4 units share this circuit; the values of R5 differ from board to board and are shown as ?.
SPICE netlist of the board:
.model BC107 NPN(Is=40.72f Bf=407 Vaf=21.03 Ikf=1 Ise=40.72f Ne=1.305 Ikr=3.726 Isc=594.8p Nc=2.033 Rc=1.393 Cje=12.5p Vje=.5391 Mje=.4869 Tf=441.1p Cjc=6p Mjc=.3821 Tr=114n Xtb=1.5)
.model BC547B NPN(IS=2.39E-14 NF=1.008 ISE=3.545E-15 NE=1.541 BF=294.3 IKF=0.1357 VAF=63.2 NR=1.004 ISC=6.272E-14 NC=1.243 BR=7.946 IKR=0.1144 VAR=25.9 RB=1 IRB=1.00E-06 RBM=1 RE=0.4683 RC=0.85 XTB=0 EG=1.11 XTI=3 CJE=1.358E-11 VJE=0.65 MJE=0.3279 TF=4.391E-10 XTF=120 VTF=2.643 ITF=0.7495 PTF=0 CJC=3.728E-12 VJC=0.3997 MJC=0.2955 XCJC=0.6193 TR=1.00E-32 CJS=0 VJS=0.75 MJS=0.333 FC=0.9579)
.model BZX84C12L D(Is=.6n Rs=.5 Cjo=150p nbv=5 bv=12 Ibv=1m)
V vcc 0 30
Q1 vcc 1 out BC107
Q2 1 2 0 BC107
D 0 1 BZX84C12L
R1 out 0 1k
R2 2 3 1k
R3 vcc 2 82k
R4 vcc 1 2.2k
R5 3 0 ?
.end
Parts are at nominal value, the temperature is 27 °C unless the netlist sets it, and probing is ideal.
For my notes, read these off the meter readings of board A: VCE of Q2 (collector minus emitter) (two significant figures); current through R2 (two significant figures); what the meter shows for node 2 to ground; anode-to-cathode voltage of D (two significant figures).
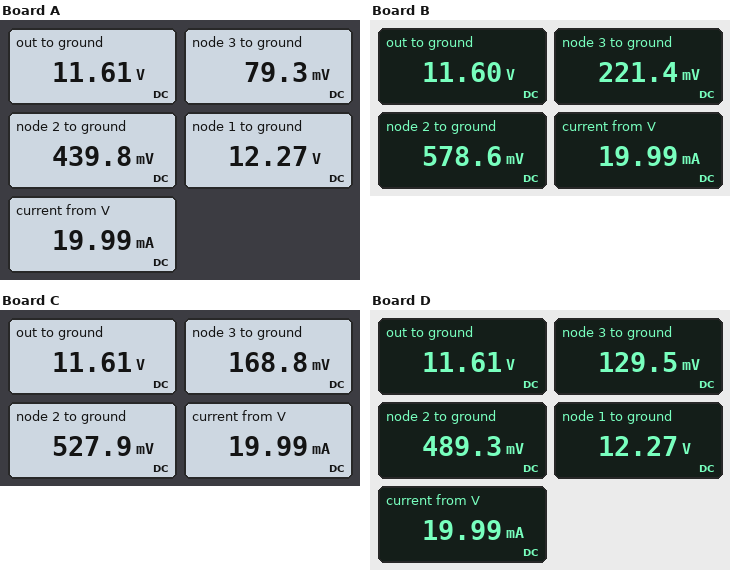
12 V
360 µA
439.8 mV
-12 V
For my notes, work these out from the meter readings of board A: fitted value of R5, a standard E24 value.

220 Ω
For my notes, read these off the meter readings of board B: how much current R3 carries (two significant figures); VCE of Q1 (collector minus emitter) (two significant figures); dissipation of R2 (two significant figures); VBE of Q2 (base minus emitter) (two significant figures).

360 µA
18 V
130 µW
580 mV
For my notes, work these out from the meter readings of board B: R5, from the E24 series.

620 Ω
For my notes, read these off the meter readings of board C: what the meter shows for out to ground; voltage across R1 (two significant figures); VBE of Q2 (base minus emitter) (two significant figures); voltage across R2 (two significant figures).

11.61 V
12 V
530 mV
360 mV
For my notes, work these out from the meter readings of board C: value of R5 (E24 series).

470 Ω
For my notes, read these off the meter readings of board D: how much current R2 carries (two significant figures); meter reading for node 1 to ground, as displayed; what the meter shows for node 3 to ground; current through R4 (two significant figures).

360 µA
12.27 V
129.5 mV
8.1 mA
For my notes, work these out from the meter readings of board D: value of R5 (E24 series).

360 Ω
